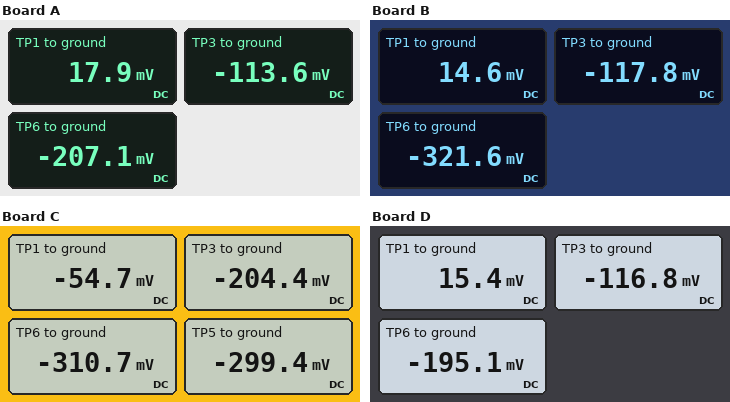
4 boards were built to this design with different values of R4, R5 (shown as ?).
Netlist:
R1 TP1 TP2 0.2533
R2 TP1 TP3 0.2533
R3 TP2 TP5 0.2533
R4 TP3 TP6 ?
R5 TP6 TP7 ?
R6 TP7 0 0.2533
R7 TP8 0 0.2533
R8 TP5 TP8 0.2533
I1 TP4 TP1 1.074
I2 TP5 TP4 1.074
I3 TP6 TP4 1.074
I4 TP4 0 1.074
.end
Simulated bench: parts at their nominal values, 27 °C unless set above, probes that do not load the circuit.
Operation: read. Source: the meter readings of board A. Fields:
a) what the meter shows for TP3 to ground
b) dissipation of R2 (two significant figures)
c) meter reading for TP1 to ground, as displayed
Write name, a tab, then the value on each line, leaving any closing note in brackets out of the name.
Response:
what the meter shows for TP3 to ground	-113.6 mV
dissipation of R2	68 mW
meter reading for TP1 to ground, as displayed	17.9 mV
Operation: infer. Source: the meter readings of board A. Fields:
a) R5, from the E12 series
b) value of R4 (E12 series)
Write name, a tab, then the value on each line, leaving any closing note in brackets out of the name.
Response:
R5, from the E12 series	0.12 Ω
value of R4	0.18 Ω
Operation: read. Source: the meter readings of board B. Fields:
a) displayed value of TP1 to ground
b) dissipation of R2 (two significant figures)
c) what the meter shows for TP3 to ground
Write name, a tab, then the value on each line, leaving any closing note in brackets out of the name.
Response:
displayed value of TP1 to ground	14.6 mV
dissipation of R2	69 mW
what the meter shows for TP3 to ground	-117.8 mV
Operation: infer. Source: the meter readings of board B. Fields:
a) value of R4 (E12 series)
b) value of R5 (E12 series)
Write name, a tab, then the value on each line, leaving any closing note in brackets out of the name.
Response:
value of R4	0.39 Ω
value of R5	0.33 Ω
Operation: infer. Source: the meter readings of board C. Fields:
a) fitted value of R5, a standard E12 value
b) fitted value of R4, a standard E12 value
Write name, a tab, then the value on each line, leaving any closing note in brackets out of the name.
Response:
fitted value of R5, a standard E12 value	0.39 Ω
fitted value of R4, a standard E12 value	0.18 Ω
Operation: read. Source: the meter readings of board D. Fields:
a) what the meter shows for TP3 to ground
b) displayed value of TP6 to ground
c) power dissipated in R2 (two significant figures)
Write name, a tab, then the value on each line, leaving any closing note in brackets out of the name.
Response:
what the meter shows for TP3 to ground	-116.8 mV
displayed value of TP6 to ground	-195.1 mV
power dissipated in R2	69 mW
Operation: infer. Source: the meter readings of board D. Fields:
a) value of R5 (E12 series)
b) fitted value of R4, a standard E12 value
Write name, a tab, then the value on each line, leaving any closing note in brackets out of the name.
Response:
value of R5	0.1 Ω
fitted value of R4, a standard E12 value	0.15 Ω
